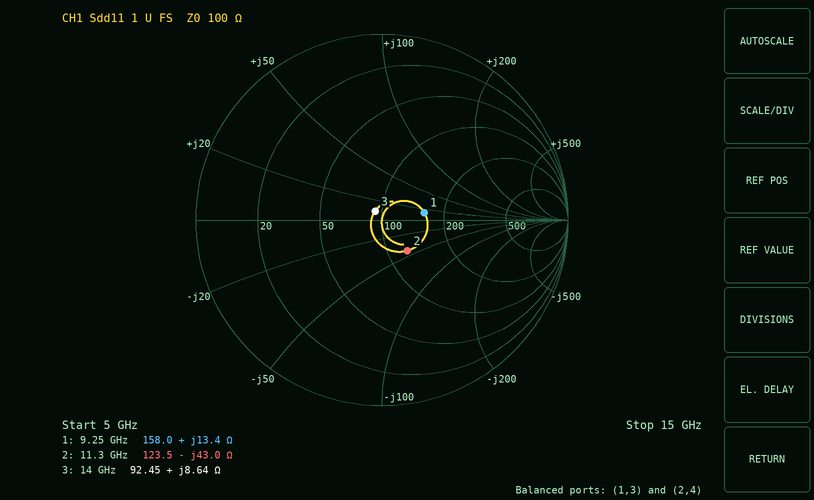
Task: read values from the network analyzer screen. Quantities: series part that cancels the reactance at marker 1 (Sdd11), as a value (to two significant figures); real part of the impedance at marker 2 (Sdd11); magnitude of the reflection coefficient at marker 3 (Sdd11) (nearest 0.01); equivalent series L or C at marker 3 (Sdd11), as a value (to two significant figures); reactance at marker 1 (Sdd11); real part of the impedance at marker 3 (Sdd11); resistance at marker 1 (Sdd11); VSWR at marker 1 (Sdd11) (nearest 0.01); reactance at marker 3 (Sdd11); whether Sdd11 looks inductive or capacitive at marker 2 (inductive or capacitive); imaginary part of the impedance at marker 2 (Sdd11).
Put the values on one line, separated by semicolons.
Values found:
1.3 pF; 123.5 Ω; 0.06; 98 pH; +13.4 Ω; 92.45 Ω; 158.0 Ω; 1.60; +8.64 Ω; capacitive; -43.0 Ω
